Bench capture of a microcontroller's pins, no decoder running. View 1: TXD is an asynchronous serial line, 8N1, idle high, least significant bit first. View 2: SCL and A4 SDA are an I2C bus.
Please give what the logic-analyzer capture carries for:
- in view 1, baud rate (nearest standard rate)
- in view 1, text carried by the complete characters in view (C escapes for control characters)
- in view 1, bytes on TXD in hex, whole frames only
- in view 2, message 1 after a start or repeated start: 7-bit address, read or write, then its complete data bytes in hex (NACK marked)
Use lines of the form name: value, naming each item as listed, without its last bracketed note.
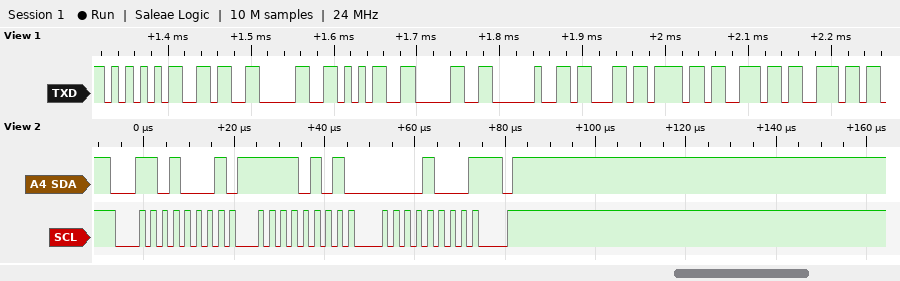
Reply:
in view 1, baud rate: 115200 baud
in view 1, text carried by the complete characters in view: "U6050 conn"
in view 1, bytes on TXD in hex, whole frames only: 55 36 30 35 30 20 63 6F 6E 6E
in view 2, message 1 after a start or repeated start: 7-bit address, read or write, then its complete data bytes in hex: 0x68 read: F5 08 NACK
